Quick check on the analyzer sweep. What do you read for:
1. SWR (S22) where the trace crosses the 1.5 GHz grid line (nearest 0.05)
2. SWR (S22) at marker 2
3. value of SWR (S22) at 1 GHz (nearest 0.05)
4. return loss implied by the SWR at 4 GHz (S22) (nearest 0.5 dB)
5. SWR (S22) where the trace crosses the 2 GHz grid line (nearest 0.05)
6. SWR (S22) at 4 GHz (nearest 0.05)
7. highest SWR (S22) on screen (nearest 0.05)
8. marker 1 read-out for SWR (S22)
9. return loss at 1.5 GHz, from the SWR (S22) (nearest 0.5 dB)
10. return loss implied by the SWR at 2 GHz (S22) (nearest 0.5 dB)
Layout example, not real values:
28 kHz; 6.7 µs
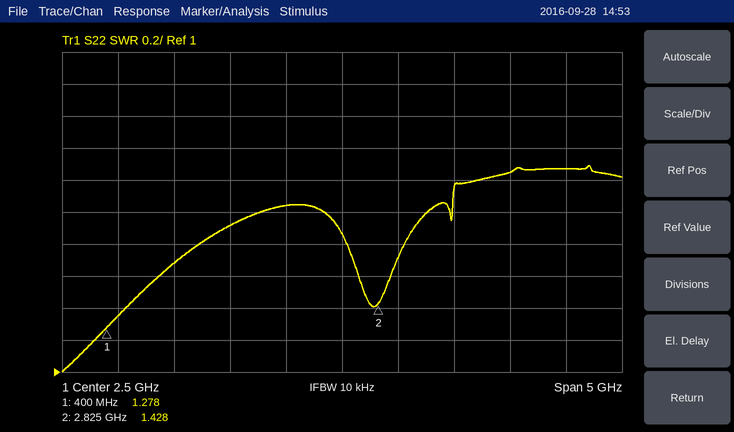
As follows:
1.90; 1.428; 1.70; 8.5 dB; 2.05; 2.25; 2.30; 1.278; 10.0 dB; 9.5 dB
